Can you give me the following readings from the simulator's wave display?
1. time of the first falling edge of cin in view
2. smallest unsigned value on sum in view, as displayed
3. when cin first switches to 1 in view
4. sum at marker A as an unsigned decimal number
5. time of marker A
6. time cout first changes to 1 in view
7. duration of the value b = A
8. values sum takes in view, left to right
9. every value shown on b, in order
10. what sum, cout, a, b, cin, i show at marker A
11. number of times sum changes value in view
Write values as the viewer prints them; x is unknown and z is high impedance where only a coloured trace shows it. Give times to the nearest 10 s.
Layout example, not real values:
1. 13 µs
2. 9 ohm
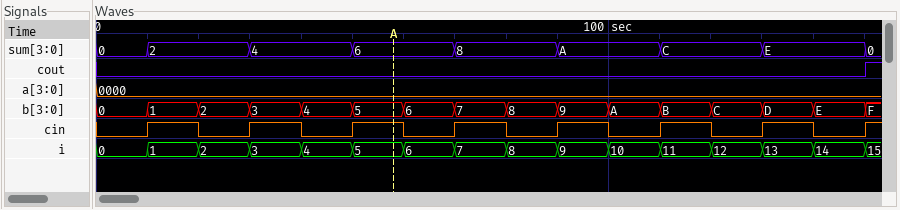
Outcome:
1. 20 s
2. 0
3. 10 s
4. 6
5. 60 s
6. 150 s
7. 10 s
8. 0, 2, 4, 6, 8, A, C, E, 0
9. 0, 1, 2, 3, 4, 5, 6, 7, 8, 9, A, B, C, D, E, F
10. sum=6, cout=0, a=0000, b=5, cin=1, i=5
11. 8
